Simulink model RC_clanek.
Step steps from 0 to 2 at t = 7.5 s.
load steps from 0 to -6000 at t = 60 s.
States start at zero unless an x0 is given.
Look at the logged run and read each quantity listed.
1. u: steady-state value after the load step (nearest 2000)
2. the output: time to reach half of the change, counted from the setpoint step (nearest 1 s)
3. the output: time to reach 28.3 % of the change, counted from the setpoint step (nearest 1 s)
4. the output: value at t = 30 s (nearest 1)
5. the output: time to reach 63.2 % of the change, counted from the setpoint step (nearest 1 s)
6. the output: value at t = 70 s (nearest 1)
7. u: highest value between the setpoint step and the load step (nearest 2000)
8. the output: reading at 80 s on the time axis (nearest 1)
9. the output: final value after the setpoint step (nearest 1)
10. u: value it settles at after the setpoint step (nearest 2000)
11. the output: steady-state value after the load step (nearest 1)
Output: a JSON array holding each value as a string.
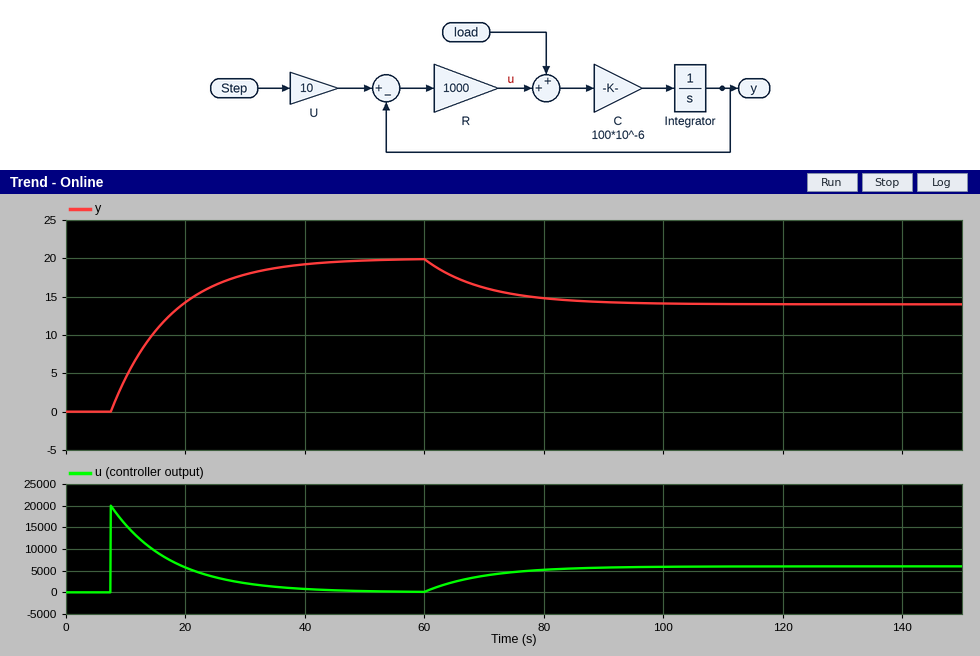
["6000", "7 s", "3 s", "18", "10 s", "16", "20000", "15", "20", "0", "14"]
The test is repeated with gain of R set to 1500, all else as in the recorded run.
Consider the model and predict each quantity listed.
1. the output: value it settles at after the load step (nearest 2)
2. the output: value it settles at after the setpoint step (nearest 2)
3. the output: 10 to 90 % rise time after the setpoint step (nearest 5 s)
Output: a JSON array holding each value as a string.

["16", "20", "15 s"]
